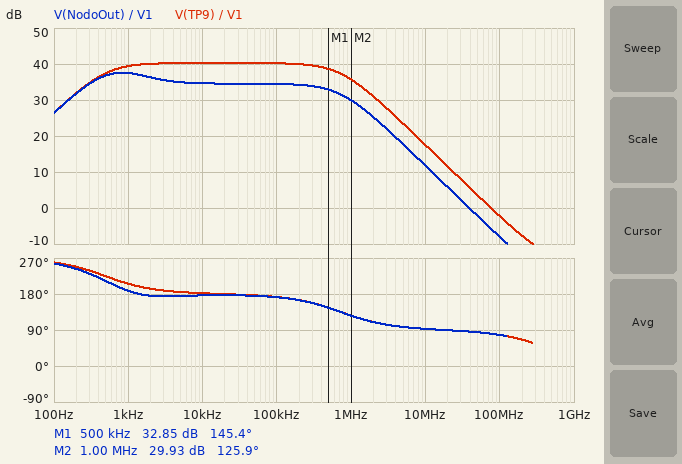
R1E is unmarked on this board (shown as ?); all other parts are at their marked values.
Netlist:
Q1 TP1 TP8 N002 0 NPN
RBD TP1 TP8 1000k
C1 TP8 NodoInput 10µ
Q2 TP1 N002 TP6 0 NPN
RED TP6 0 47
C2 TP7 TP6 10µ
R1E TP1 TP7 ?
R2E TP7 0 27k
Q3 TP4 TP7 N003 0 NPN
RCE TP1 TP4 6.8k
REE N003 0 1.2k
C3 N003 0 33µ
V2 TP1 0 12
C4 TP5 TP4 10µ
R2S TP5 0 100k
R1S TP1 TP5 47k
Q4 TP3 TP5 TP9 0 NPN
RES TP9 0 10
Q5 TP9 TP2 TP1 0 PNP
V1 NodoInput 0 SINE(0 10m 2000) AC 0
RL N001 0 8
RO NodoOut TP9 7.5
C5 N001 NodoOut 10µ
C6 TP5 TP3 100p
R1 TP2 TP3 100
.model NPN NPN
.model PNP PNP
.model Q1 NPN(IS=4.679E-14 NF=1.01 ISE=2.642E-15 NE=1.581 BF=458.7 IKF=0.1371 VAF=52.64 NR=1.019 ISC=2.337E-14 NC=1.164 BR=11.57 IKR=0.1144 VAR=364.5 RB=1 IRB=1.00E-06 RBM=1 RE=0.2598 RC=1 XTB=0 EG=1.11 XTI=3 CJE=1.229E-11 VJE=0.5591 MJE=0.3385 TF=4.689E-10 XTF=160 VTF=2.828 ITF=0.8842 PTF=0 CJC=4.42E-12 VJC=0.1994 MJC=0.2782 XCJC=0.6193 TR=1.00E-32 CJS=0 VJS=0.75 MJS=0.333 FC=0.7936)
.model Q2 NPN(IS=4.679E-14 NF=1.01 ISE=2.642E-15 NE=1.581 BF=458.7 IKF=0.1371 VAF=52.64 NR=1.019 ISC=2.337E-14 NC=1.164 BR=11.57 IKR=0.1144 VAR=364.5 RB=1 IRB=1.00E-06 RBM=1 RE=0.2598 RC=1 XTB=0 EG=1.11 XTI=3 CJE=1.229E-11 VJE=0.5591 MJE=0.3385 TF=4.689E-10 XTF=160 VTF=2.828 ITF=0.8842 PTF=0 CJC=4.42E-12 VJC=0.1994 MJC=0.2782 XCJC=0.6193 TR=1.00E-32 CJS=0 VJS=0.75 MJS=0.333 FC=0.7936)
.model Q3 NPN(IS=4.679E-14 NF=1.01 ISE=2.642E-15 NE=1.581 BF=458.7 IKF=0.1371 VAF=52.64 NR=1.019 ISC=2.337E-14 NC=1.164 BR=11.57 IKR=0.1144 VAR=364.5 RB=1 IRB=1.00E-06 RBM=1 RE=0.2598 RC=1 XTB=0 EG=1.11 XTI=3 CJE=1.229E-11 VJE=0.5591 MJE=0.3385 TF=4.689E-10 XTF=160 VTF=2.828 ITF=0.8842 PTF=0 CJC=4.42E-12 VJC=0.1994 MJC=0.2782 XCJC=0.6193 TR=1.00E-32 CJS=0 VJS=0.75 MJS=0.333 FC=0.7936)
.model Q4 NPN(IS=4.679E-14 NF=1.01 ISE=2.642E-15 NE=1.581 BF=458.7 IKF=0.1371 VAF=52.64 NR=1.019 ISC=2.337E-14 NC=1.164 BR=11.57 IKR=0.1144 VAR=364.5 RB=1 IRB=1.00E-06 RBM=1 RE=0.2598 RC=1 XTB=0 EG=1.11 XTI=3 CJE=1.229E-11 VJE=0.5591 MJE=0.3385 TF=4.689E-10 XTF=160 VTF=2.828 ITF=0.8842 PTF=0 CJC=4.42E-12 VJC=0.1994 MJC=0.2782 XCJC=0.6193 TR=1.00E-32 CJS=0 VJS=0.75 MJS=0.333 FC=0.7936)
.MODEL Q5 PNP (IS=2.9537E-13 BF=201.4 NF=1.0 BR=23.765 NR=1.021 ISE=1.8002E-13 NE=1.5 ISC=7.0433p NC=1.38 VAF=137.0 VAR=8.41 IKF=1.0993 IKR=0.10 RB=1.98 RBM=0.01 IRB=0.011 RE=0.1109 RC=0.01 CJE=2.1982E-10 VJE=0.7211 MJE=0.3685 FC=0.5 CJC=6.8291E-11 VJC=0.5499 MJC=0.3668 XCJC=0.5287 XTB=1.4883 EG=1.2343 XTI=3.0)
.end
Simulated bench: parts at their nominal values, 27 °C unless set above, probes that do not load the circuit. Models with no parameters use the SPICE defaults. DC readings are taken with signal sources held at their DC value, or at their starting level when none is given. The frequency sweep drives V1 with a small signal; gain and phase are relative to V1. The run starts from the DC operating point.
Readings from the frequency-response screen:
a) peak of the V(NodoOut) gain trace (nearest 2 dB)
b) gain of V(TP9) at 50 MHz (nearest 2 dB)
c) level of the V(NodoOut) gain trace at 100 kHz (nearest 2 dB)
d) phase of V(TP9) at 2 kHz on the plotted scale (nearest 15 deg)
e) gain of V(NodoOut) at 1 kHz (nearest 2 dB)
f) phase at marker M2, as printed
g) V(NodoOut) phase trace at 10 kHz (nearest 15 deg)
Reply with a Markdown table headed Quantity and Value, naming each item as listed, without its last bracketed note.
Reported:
| Quantity | Value |
|---|---|
| peak of the V(NodoOut) gain trace | 38 dB |
| gain of V(TP9) at 50 MHz | 4 dB |
| level of the V(NodoOut) gain trace at 100 kHz | 34 dB |
| phase of V(TP9) at 2 kHz on the plotted scale | 195 deg |
| gain of V(NodoOut) at 1 kHz | 38 dB |
| phase at marker M2, as printed | 125.9 deg |
| V(NodoOut) phase trace at 10 kHz | 180 deg |
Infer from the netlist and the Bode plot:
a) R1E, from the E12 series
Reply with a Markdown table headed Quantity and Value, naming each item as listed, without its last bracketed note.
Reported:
| Quantity | Value |
|---|---|
| R1E, from the E12 series | 82 kΩ |
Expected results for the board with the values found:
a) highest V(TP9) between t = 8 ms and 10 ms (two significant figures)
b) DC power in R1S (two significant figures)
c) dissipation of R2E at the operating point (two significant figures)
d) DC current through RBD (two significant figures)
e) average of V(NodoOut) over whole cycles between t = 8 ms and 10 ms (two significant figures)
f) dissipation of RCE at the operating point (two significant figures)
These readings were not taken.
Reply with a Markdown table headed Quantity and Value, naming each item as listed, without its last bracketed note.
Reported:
| Quantity | Value |
|---|---|
| highest V(TP9) between t = 8 ms and 10 ms | 8.5 V |
| DC power in R1S | 670 µW |
| dissipation of R2E at the operating point | 250 µW |
| DC current through RBD | 7.0 µA |
| average of V(NodoOut) over whole cycles between t = 8 ms and 10 ms | 6.7 V |
| dissipation of RCE at the operating point | 15 mW |
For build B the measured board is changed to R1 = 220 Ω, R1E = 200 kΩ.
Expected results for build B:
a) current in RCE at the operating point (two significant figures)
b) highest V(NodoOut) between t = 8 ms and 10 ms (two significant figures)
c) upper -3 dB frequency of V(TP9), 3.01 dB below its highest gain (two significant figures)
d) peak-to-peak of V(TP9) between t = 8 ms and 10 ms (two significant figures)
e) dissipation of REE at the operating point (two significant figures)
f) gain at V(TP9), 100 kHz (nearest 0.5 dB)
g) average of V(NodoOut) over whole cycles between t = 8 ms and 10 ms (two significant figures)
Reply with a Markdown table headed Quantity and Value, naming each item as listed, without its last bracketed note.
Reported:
| Quantity | Value |
|---|---|
| current in RCE at the operating point | 460 µA |
| highest V(NodoOut) between t = 8 ms and 10 ms | 6.1 V |
| upper -3 dB frequency of V(TP9), 3.01 dB below its highest gain | 220 kHz |
| peak-to-peak of V(TP9) between t = 8 ms and 10 ms | 1.8 V |
| dissipation of REE at the operating point | 260 µW |
| gain at V(TP9), 100 kHz | 38.5 dB |
| average of V(NodoOut) over whole cycles between t = 8 ms and 10 ms | 5.6 V |
